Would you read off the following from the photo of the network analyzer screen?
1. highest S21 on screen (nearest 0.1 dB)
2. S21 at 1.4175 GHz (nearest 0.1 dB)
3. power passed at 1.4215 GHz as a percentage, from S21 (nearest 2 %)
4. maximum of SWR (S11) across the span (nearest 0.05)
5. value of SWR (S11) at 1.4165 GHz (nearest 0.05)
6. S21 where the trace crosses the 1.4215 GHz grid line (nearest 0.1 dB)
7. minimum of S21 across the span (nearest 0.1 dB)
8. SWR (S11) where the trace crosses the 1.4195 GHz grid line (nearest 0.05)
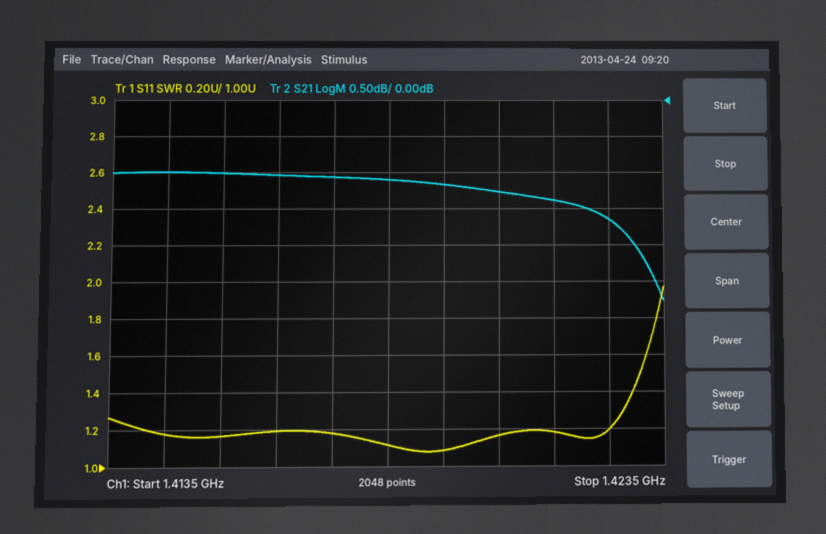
-1.0 dB
-1.1 dB
72 %
1.95
1.20
-1.4 dB
-2.8 dB
1.10
